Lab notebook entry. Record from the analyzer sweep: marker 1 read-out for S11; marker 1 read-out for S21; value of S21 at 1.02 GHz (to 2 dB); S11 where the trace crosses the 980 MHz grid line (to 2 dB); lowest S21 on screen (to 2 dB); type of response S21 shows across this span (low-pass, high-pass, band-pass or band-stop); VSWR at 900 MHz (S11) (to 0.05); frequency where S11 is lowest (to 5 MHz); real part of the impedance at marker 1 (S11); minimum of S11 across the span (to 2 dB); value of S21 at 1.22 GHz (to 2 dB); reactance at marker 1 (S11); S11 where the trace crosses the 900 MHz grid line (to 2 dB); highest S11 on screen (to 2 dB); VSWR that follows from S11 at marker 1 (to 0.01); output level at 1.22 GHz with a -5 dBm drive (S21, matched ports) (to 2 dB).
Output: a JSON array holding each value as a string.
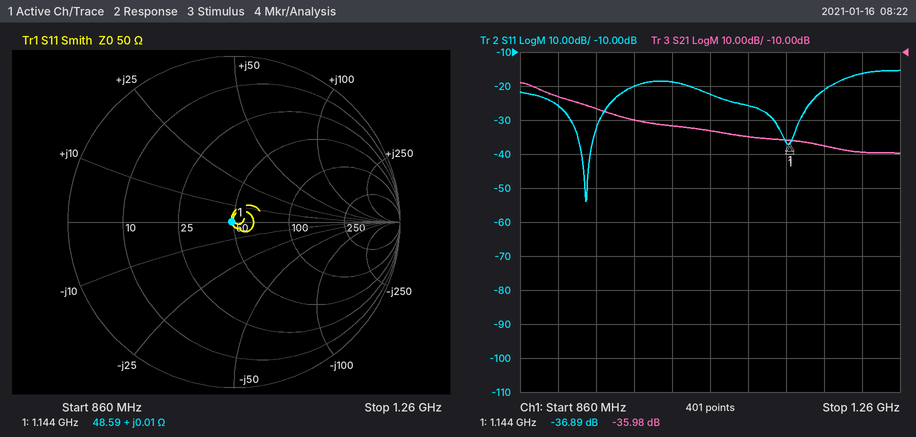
["-36.89 dB", "-35.98 dB", "-32 dB", "-20 dB", "-40 dB", "low-pass", "1.10", "930 MHz", "48.59 Ω", "-54 dB", "-40 dB", "+0.01 Ω", "-26 dB", "-16 dB", "1.03", "-44 dBm"]
